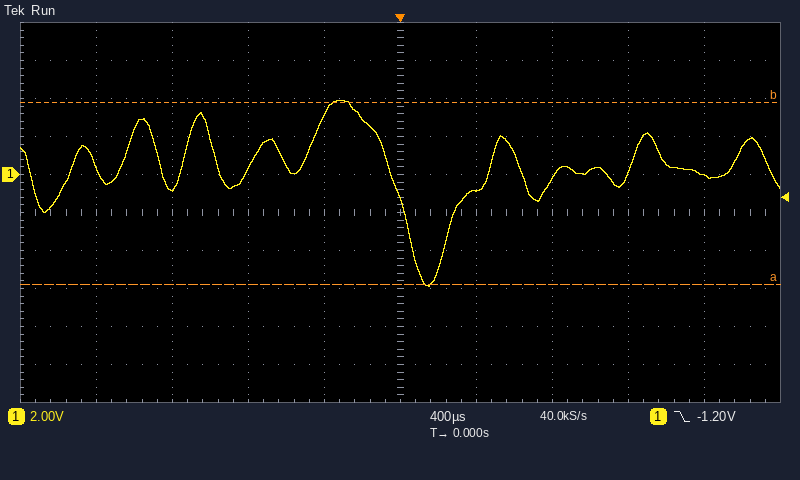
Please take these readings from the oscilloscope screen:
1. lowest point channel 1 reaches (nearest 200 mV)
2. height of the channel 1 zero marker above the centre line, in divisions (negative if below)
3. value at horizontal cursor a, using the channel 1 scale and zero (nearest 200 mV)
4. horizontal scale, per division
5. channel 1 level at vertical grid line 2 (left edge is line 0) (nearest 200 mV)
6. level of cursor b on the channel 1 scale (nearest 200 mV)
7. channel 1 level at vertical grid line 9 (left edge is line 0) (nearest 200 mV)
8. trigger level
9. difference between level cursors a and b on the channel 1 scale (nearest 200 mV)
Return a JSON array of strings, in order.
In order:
["-5.8 V", "+1.0 div", "-5.8 V", "400 µs", "-800 mV", "3.8 V", "0.0 V", "-1.20 V", "9.6 V"]
